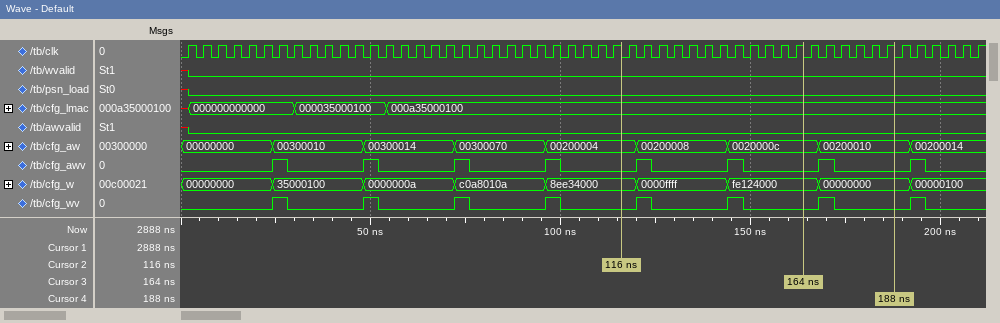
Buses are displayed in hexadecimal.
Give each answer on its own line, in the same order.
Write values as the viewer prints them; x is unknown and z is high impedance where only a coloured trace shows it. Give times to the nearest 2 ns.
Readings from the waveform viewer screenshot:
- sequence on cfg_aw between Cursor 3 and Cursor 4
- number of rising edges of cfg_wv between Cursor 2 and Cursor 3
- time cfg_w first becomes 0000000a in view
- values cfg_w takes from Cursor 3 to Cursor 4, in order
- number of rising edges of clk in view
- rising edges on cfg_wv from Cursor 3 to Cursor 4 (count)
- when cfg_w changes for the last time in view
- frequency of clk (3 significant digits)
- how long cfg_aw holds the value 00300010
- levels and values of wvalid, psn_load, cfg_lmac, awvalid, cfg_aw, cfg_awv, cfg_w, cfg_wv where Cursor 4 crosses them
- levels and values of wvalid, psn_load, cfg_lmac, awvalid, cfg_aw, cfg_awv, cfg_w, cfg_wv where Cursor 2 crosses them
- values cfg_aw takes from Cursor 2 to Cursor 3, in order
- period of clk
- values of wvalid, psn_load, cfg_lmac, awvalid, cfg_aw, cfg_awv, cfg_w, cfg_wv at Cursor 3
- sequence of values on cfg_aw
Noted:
0020000c, 00200010
2
48 ns
fe124000, 00000000
53
1
192 ns
250 MHz
24 ns
wvalid=0, psn_load=0, cfg_lmac=000a35000100, awvalid=0, cfg_aw=00200010, cfg_awv=0, cfg_w=00000000, cfg_wv=0
wvalid=0, psn_load=0, cfg_lmac=000a35000100, awvalid=0, cfg_aw=00200004, cfg_awv=0, cfg_w=8ee34000, cfg_wv=0
00200004, 00200008, 0020000c
4 ns
wvalid=0, psn_load=0, cfg_lmac=000a35000100, awvalid=0, cfg_aw=0020000c, cfg_awv=0, cfg_w=fe124000, cfg_wv=0
00000000, 00300010, 00300014, 00300070, 00200004, 00200008, 0020000c, 00200010, 00200014
